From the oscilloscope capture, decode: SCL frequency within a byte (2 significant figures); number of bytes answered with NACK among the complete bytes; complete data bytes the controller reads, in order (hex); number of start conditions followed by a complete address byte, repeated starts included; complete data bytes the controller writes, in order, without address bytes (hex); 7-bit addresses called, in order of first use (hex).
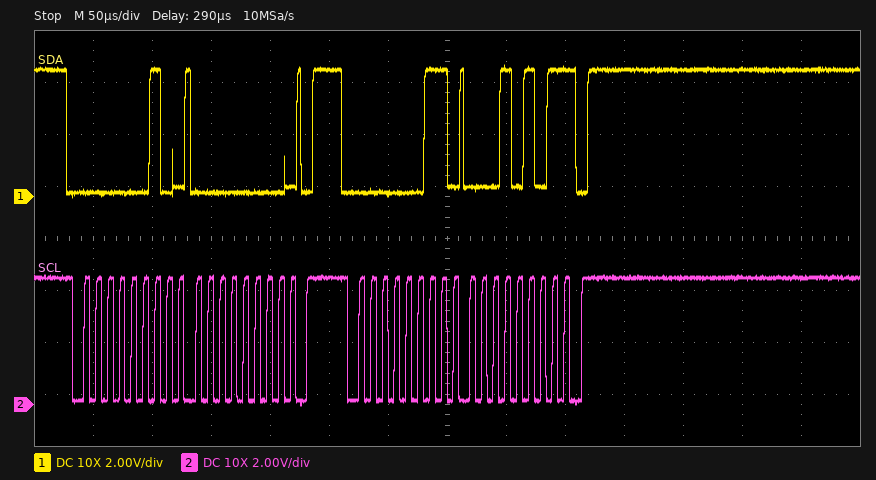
100 kHz
1
15
2
00
0x01
